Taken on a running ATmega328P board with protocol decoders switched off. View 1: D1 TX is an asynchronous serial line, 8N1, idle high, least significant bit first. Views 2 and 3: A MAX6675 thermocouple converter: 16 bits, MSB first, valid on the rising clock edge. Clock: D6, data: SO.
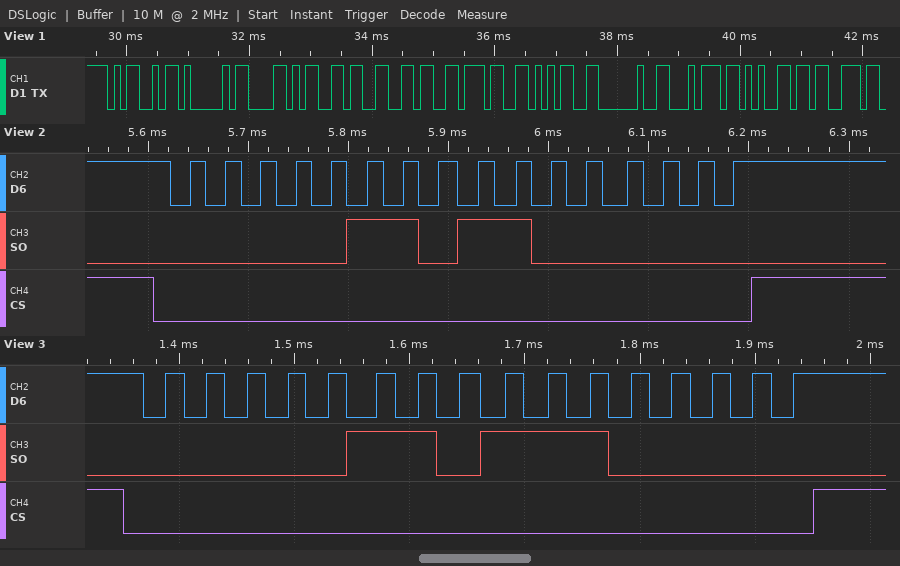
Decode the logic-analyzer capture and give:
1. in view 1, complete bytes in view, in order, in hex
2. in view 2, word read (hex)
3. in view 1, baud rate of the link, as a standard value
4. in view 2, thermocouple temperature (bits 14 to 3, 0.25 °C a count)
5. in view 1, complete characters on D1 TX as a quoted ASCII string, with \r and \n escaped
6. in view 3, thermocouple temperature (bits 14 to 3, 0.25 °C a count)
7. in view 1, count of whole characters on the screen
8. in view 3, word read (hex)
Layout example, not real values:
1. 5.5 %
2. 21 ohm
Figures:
1. 0x4D 0x41 0x58 0x36 0x36 0x37 0x35 0x20 0x74 0x65 0x73
2. 0x06C0
3. 9600 baud
4. 54.00 °C
5. "MAX6675 tes"
6. 55.00 °C
7. 11
8. 0x06E0
